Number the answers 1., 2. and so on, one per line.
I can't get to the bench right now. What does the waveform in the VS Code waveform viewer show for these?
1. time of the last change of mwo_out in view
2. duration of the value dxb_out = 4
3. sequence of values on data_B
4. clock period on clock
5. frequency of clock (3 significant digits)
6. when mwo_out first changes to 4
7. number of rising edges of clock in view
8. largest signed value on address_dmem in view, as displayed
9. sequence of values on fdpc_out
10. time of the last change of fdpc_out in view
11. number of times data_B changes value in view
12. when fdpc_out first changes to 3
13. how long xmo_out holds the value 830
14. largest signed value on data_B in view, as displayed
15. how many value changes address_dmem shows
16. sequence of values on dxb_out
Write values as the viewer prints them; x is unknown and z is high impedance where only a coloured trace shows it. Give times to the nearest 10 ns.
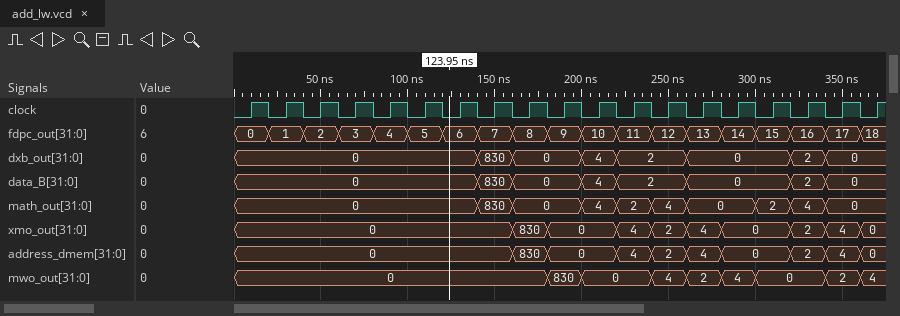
1. 360 ns
2. 20 ns
3. 0, 830, 0, 4, 2, 0, 2, 0
4. 20 ns
5. 50.0 MHz
6. 240 ns
7. 19
8. 830
9. 0, 1, 2, 3, 4, 5, 6, 7, 8, 9, 10, 11, 12, 13, 14, 15, 16, 17, 18
10. 360 ns
11. 7
12. 60 ns
13. 20 ns
14. 830
15. 9
16. 0, 830, 0, 4, 2, 0, 2, 0
